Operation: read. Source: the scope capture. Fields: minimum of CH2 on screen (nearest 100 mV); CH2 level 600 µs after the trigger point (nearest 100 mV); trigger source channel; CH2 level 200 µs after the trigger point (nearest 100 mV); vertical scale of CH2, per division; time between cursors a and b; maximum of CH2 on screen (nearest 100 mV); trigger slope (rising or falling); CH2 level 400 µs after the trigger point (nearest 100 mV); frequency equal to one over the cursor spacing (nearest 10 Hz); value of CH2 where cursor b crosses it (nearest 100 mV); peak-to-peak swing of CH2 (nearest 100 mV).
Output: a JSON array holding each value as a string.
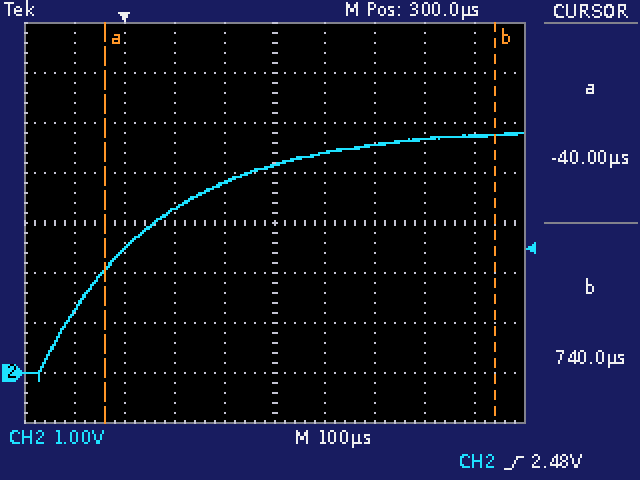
["-200 mV", "4.7 V", "CH2", "3.8 V", "1 V", "780 µs", "4.8 V", "rising", "4.4 V", "1.28 kHz", "4.8 V", "5.0 V"]
